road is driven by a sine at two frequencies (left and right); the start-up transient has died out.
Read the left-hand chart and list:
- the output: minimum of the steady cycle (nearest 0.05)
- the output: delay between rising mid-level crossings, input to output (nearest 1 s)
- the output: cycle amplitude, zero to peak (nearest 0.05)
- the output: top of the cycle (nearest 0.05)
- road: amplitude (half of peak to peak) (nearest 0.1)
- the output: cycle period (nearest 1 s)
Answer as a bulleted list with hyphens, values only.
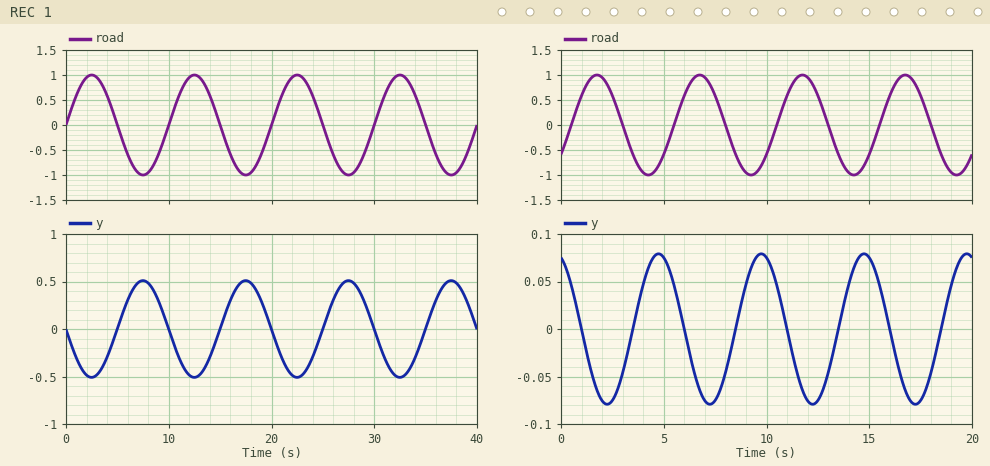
- -0.50
- 5 s
- 0.50
- 0.50
- 1.0
- 10 s
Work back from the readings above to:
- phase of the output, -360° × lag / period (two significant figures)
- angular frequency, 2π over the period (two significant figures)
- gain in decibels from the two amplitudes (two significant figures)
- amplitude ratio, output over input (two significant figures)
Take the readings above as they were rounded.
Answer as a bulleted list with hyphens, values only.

- -180°
- 0.63 rad/s
- -6.0 dB
- 0.50
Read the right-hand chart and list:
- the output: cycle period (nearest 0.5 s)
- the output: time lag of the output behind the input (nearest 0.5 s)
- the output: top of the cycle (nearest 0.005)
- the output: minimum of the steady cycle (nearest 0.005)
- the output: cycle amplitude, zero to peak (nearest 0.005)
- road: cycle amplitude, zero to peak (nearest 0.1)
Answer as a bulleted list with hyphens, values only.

- 5.0 s
- 3.0 s
- 0.080
- -0.080
- 0.080
- 1.0
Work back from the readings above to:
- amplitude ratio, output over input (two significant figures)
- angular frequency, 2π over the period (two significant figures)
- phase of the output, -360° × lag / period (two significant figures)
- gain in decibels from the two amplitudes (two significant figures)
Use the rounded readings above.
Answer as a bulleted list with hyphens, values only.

- 0.080
- 1.3 rad/s
- -220°
- -22 dB
